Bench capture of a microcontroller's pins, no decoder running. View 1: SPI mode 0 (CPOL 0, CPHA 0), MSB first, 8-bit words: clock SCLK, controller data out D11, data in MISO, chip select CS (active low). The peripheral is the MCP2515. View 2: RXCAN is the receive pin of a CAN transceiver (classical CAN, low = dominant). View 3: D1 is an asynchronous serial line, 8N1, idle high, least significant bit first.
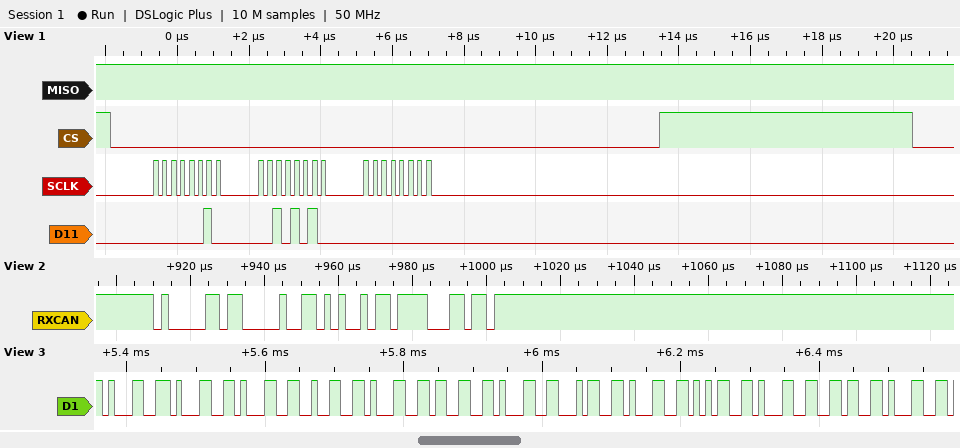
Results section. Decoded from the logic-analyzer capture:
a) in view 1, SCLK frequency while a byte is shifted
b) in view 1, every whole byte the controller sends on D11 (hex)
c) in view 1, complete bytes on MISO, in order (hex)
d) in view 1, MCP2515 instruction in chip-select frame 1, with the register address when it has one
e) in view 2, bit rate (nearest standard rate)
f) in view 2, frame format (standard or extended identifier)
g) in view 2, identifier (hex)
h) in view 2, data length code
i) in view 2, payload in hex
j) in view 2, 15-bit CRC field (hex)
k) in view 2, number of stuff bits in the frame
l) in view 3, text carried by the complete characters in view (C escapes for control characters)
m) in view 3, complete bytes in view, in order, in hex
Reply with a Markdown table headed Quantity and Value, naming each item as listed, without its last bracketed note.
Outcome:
| Quantity | Value |
|---|---|
| in view 1, SCLK frequency while a byte is shifted | 4 MHz |
| in view 1, every whole byte the controller sends on D11 | 02 2A 00 |
| in view 1, complete bytes on MISO, in order | FF FF FF |
| in view 1, MCP2515 instruction in chip-select frame 1, with the register address when it has one | WRITE 0x2A |
| in view 2, bit rate | 500 kbit/s |
| in view 2, frame format | standard |
| in view 2, identifier | 0x416 |
| in view 2, data length code | 1 |
| in view 2, payload in hex | A9 |
| in view 2, 15-bit CRC field | 0x378D |
| in view 2, number of stuff bits in the frame | 2 |
| in view 3, text carried by the complete characters in view | "1112131415161" |
| in view 3, complete bytes in view, in order, in hex | 31 31 31 32 31 33 31 34 31 35 31 36 31 |
